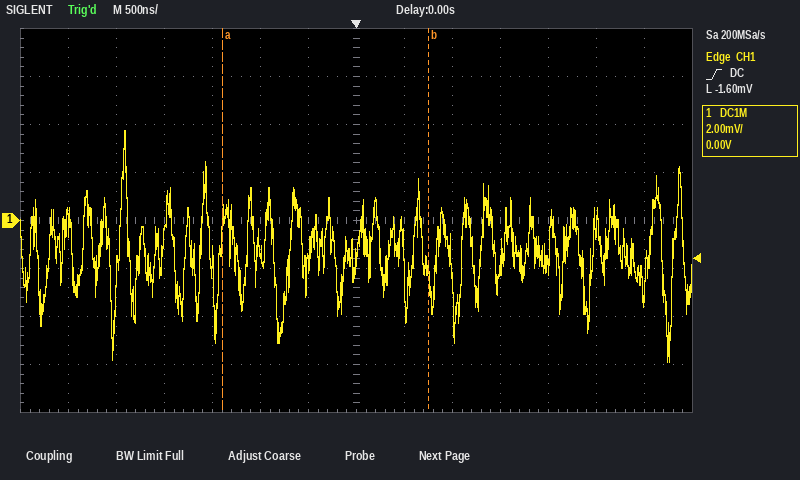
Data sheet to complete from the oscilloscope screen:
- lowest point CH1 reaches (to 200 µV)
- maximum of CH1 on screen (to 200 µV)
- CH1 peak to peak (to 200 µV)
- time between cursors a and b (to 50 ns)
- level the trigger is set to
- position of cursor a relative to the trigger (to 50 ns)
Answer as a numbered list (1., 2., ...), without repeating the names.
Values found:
1. -5.8 mV
2. 3.8 mV
3. 9.6 mV
4. 2.15 µs
5. -1.60 mV
6. -1.40 µs
